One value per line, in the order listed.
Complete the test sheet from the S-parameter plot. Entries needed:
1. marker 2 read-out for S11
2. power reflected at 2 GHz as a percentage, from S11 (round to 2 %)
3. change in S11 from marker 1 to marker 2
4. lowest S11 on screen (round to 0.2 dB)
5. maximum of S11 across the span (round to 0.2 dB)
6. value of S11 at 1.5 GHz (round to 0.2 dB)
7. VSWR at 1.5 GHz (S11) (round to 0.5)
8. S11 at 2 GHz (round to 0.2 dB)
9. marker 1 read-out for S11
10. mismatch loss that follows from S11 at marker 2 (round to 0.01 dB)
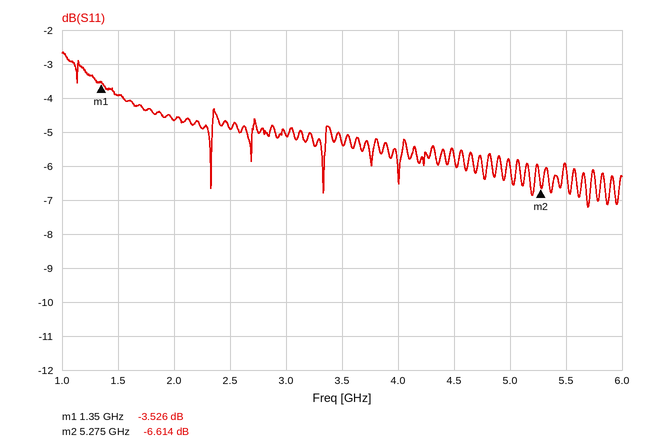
-6.614 dB
34 %
-3.088 dB
-7.2 dB
-2.6 dB
-4.0 dB
4.5
-4.6 dB
-3.526 dB
1.07 dB
